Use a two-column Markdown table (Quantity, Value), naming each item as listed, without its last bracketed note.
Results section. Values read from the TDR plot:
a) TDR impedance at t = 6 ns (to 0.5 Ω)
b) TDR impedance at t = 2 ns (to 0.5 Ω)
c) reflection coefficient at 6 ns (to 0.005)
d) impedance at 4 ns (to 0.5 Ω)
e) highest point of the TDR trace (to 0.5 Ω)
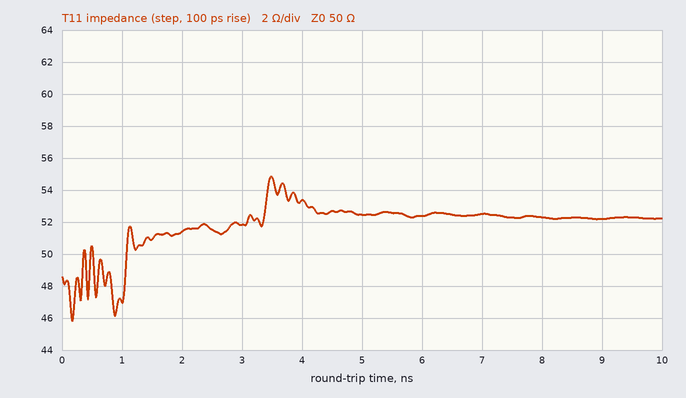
| Quantity | Value |
|---|---|
| TDR impedance at t = 6 ns | 52.5 Ω |
| TDR impedance at t = 2 ns | 51.5 Ω |
| reflection coefficient at 6 ns | +0.025 |
| impedance at 4 ns | 53.5 Ω |
| highest point of the TDR trace | 55.0 Ω |
